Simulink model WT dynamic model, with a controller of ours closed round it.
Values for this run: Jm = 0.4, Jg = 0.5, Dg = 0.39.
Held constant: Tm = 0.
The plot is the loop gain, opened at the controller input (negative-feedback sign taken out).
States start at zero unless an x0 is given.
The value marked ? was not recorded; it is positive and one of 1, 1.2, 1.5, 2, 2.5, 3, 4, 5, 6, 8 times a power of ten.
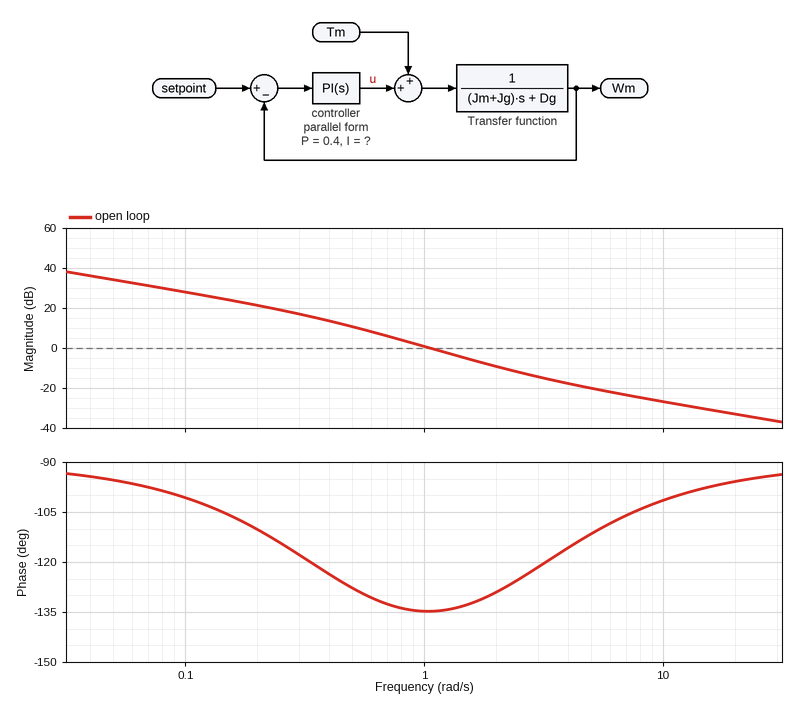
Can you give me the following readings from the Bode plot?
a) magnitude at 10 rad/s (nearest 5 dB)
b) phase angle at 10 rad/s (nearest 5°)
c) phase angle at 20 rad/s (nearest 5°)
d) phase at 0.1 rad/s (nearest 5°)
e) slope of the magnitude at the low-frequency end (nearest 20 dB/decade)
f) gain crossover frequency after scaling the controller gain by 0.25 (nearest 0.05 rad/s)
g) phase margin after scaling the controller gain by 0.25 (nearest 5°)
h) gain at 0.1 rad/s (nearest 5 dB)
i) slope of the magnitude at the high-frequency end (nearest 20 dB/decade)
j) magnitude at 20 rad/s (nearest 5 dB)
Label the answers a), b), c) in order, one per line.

a) -25 dB
b) -100°
c) -95°
d) -100°
e) -20 dB/decade
f) 0.45 rad/s
g) 55°
h) 30 dB
i) -20 dB/decade
j) -35 dB
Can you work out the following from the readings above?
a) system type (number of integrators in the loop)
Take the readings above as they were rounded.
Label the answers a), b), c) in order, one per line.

a) 1
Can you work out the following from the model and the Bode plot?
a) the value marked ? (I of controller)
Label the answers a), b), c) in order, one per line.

a) 1
